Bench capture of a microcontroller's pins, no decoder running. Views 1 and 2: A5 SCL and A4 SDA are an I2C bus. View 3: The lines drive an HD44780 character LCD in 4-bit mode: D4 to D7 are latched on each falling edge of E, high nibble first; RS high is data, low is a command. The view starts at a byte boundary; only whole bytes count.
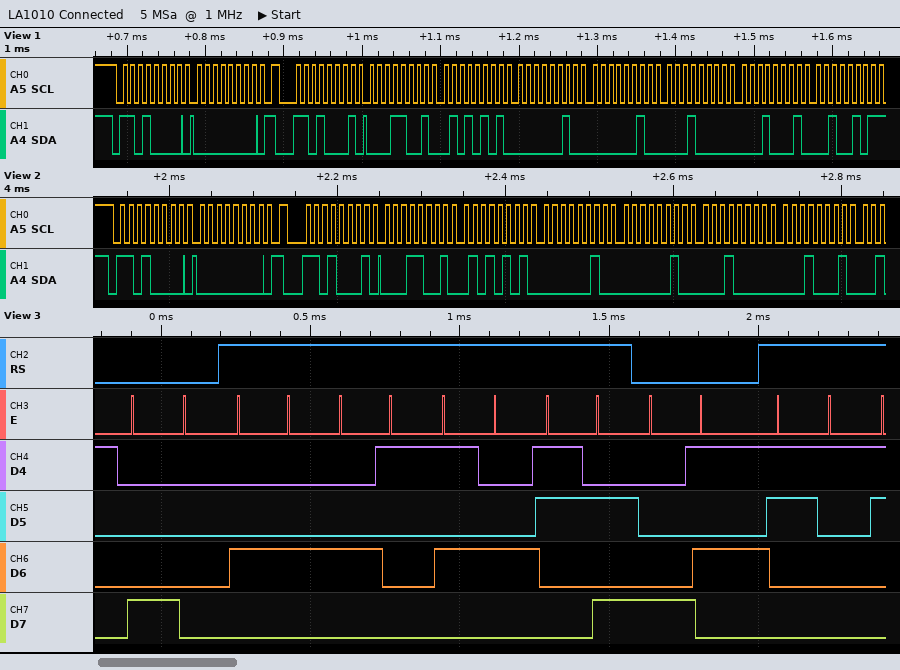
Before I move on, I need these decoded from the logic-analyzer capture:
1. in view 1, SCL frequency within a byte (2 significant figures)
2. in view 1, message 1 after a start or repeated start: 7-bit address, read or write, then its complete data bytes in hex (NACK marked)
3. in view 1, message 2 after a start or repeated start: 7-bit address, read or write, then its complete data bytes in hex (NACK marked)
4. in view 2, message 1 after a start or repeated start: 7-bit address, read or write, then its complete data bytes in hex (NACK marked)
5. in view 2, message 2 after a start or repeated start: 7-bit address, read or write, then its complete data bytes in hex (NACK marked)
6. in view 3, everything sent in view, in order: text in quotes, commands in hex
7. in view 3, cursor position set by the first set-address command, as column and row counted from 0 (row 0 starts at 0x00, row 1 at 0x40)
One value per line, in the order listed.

100 kHz
0x68 write: 00
0x68 read: 19 55 02 02 10 11 25 NACK
0x68 write: 00
0x68 read: 19 55 02 02 10 11
0x80 "DAT:" 0x85 "1"
column 0, row 0
